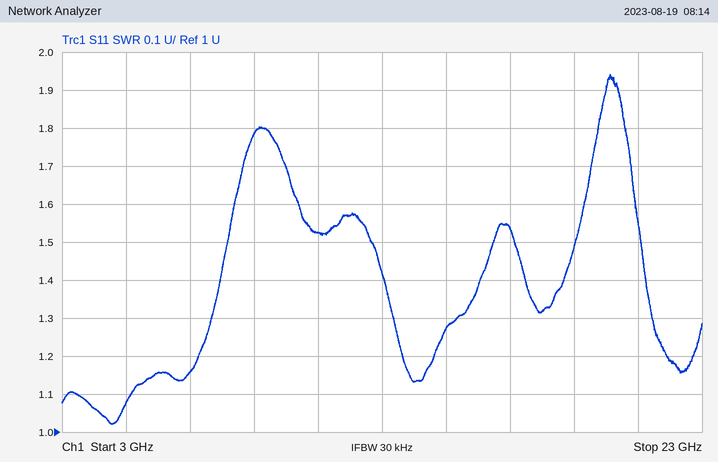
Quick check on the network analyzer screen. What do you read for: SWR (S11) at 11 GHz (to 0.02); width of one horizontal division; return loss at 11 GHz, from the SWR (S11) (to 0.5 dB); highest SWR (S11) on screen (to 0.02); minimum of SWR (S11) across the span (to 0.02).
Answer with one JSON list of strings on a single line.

["1.52", "2 GHz", "13.5 dB", "1.94", "1.02"]
